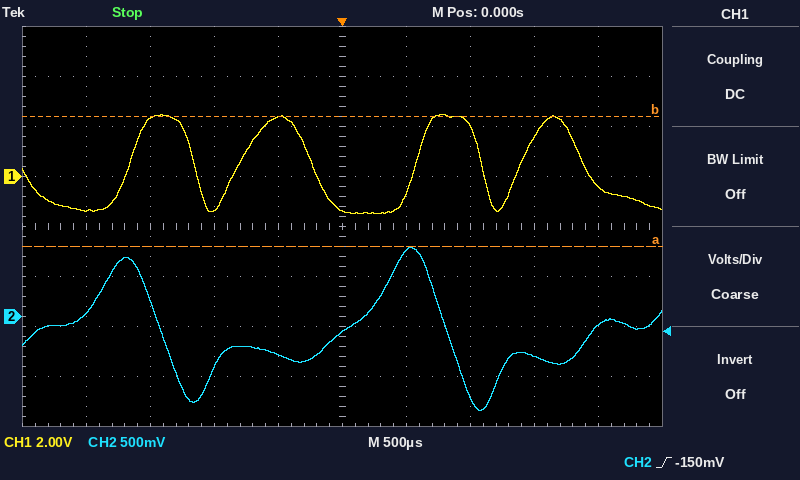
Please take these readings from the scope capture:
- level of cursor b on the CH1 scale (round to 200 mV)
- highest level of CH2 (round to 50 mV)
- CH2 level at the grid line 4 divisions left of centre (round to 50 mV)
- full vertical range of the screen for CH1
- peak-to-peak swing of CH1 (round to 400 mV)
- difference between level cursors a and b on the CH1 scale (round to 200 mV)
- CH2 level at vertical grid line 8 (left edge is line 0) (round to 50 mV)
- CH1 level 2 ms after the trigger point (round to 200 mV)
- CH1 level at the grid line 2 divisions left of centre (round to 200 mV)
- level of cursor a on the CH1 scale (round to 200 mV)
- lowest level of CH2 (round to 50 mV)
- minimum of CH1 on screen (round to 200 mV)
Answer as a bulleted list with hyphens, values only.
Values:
- 2.4 V
- 700 mV
- 50 mV
- 16 V
- 4.0 V
- 5.2 V
- -400 mV
- -400 mV
- -1.4 V
- -2.8 V
- -950 mV
- -1.4 V
